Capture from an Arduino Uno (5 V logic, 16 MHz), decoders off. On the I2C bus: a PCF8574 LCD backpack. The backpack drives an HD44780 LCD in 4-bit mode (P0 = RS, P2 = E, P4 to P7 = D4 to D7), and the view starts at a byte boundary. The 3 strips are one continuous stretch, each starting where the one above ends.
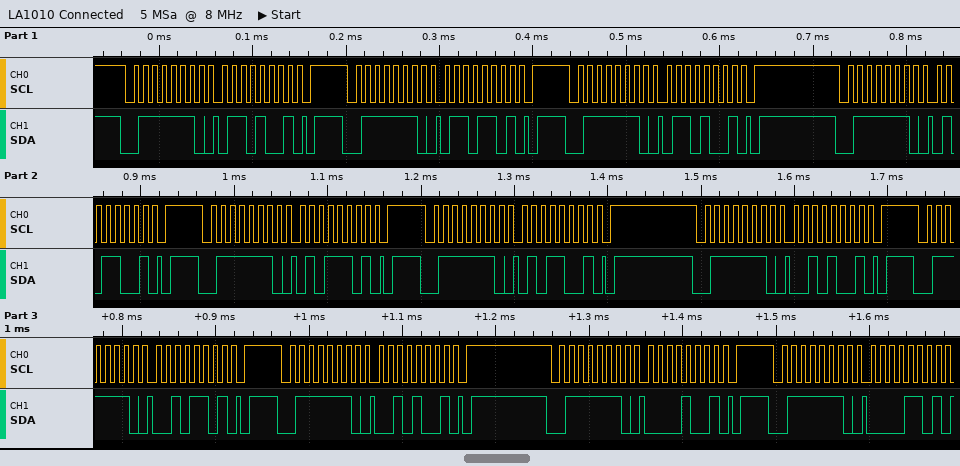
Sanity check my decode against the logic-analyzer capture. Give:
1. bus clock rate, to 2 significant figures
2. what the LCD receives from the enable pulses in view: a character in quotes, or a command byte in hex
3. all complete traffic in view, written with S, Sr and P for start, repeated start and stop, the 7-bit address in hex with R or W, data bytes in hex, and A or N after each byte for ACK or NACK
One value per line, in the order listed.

100 kHz
'e'
S 3FW A 69 A P S 3FW A 6D A P S 3FW A 69 A P S 3FW A 59 A P S 3FW A 5D A P S 3FW A 59 A P S 3FW A 29 A P S 3FW A 2D A P S 3FW A 29 A P S 3FW A 09 A P S 3FW A 0D A
